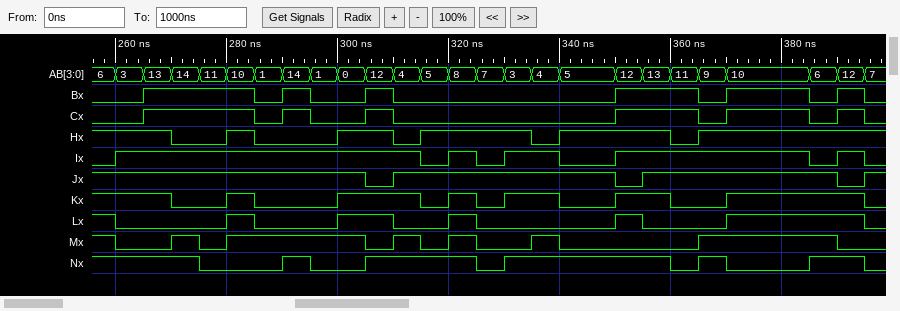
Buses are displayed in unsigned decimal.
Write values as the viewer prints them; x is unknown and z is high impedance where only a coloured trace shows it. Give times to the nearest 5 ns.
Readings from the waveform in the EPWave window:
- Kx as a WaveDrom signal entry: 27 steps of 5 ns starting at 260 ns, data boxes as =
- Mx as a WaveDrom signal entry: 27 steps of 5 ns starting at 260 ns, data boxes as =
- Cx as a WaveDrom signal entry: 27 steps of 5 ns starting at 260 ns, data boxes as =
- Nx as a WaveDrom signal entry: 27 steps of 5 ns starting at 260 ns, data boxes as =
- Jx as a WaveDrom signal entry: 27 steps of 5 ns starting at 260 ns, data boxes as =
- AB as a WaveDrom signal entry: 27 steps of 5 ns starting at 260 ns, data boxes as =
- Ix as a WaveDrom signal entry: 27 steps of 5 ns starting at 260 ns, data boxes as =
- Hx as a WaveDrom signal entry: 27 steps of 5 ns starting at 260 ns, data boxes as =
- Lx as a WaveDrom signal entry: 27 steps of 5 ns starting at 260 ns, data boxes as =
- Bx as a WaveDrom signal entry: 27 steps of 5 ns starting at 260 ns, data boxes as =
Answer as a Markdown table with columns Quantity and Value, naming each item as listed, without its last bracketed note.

| Quantity | Value |
|---|---|
| Kx as a WaveDrom signal entry: 27 steps of 5 ns starting at 260 ns, data boxes as = | {name: 'Kx', wave: '1.0.10..1..0101.0.1.0.1....'} |
| Mx as a WaveDrom signal entry: 27 steps of 5 ns starting at 260 ns, data boxes as = | {name: 'Mx', wave: '0.101....01010.10....1....0'} |
| Cx as a WaveDrom signal entry: 27 steps of 5 ns starting at 260 ns, data boxes as = | {name: 'Cx', wave: '01...010.10.......1..01..01'} |
| Nx as a WaveDrom signal entry: 27 steps of 5 ns starting at 260 ns, data boxes as = | {name: 'Nx', wave: '1..0..10.1...01.....010..1.'} |
| Jx as a WaveDrom signal entry: 27 steps of 5 ns starting at 260 ns, data boxes as = | {name: 'Jx', wave: '1........01.......01......0'} |
| AB as a WaveDrom signal entry: 27 steps of 5 ns starting at 260 ns, data boxes as = | {name: 'AB', wave: '=================.=====..==', data: '3 13 14 11 10 1 14 1 0 12 4 5 8 7 3 4 5 12 13 11 9 10 6 12'} |
| Ix as a WaveDrom signal entry: 27 steps of 5 ns starting at 260 ns, data boxes as = | {name: 'Ix', wave: '1..........0101.0.1......01'} |
| Hx as a WaveDrom signal entry: 27 steps of 5 ns starting at 260 ns, data boxes as = | {name: 'Hx', wave: '1.0.10..1.01...01...01.....'} |
| Lx as a WaveDrom signal entry: 27 steps of 5 ns starting at 260 ns, data boxes as = | {name: 'Lx', wave: '0...10..1.0.10....10..1....'} |
| Bx as a WaveDrom signal entry: 27 steps of 5 ns starting at 260 ns, data boxes as = | {name: 'Bx', wave: '01...010.10.......1..01..01'} |
